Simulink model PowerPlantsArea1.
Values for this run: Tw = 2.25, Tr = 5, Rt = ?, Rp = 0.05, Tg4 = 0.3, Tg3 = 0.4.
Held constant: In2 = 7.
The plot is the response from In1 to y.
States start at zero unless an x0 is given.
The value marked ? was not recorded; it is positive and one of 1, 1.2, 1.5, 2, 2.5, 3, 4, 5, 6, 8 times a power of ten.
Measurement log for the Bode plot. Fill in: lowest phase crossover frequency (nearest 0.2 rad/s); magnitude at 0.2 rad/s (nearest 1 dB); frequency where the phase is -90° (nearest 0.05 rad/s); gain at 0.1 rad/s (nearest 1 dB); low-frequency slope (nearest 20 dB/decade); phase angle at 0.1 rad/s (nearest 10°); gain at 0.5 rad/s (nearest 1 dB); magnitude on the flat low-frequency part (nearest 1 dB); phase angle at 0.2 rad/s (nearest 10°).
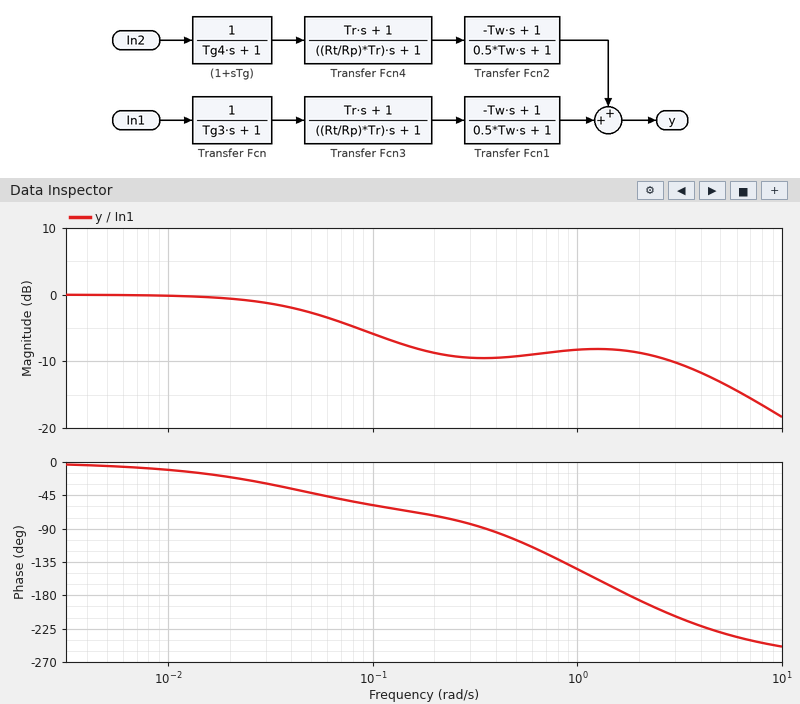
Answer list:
1.8 rad/s
-9 dB
0.35 rad/s
-6 dB
0 dB/decade
-60°
-9 dB
0 dB
-70°
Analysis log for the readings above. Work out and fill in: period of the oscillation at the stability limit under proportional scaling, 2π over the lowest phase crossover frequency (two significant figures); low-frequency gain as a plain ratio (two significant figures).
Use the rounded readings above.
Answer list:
3.5 s
1.0
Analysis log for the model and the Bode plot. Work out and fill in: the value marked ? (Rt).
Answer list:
0.2
